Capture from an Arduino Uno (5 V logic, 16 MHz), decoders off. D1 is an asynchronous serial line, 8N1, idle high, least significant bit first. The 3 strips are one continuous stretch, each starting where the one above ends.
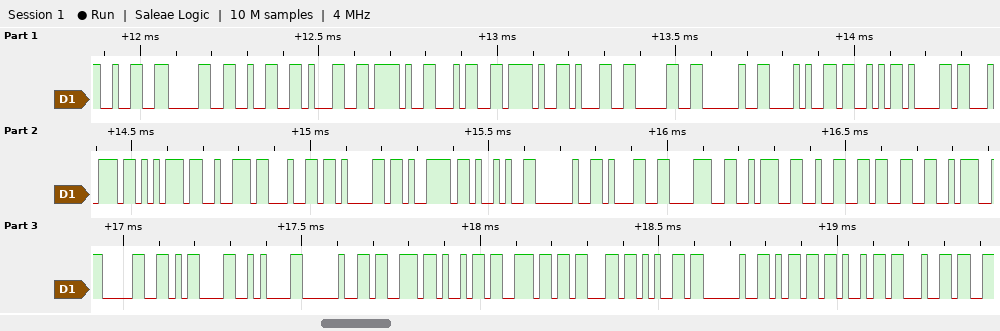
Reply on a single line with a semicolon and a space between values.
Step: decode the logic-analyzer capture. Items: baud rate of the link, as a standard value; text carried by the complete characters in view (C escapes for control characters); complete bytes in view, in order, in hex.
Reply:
57600 baud; "2021/4/10 (Saturday) 18:23:0\r\n since mid"; 32 30 32 31 2F 34 2F 31 30 20 28 53 61 74 75 72 64 61 79 29 20 31 38 3A 32 33 3A 30 0D 0A 20 73 69 6E 63 65 20 6D 69 64
